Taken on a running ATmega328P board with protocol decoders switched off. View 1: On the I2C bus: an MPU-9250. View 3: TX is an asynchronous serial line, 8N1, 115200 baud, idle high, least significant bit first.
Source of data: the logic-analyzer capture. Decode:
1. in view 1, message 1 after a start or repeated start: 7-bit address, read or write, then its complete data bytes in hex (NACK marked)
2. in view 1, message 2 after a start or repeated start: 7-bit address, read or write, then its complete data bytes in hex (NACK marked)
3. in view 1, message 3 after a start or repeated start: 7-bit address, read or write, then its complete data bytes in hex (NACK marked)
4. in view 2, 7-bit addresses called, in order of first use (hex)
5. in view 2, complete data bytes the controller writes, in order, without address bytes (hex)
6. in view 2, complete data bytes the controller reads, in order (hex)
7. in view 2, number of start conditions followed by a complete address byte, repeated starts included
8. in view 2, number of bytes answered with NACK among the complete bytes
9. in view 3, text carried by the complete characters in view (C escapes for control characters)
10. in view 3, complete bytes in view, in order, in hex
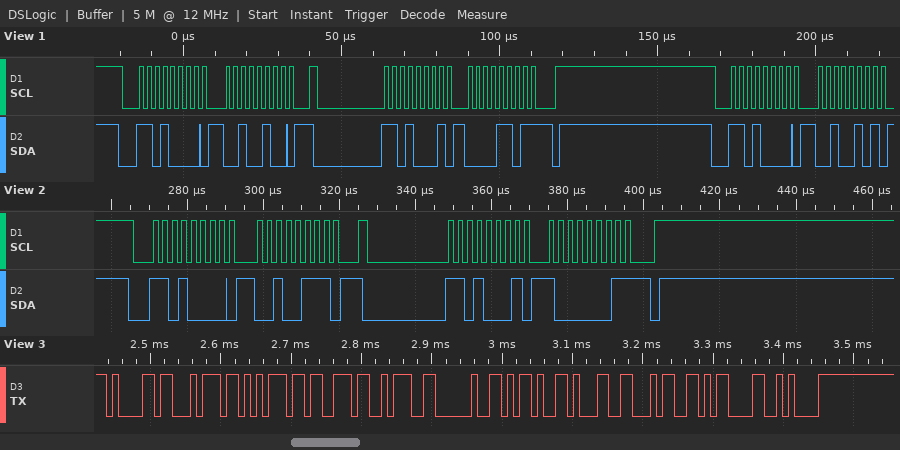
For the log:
0x68 write: 24
0x68 read: 0D NACK
0x68 write: 25
0x68
27
81
2
1
"atus: -14\r\n"
61 74 75 73 3A 20 2D 31 34 0D 0A
